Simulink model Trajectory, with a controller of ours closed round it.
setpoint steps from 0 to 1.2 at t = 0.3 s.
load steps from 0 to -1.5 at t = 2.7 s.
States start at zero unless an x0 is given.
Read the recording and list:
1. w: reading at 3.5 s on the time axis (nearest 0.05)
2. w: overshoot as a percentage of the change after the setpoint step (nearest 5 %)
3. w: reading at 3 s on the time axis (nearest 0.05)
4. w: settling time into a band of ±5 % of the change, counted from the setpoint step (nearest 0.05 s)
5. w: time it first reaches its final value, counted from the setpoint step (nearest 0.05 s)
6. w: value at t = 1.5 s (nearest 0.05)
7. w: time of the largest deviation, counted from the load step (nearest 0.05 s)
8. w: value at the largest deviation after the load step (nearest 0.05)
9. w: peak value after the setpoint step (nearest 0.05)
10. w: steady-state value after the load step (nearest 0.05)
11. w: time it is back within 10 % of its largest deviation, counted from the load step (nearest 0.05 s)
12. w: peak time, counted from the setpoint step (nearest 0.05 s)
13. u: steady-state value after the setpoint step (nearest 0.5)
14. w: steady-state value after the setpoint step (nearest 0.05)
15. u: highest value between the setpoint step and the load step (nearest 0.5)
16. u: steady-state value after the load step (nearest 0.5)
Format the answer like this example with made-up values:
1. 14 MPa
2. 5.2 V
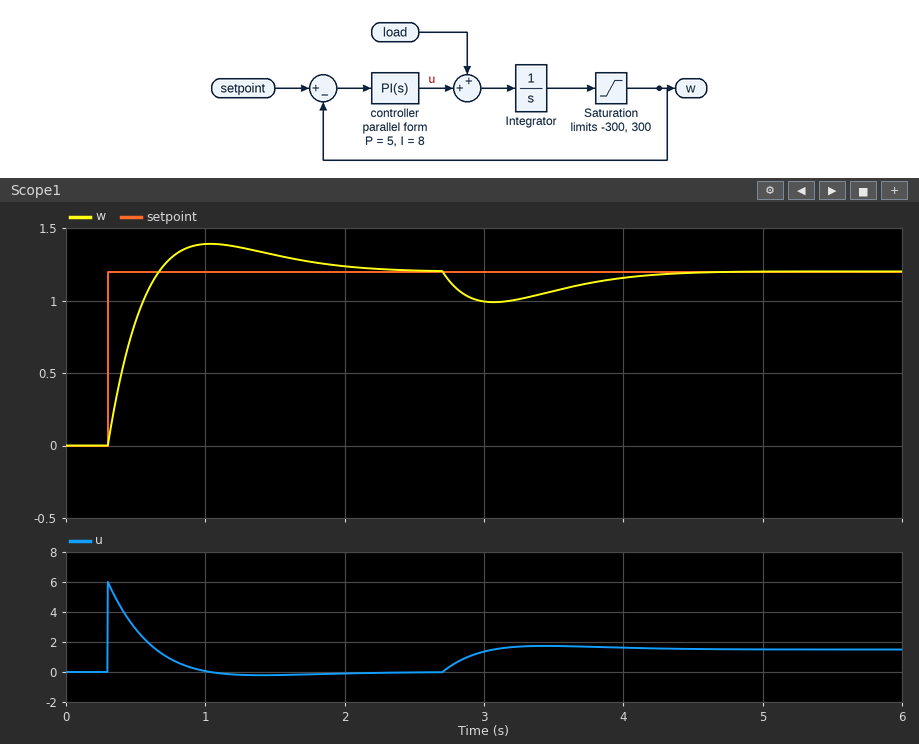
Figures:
1. 1.05
2. 15 %
3. 1.00
4. 1.50 s
5. 0.35 s
6. 1.30
7. 0.35 s
8. 1.00
9. 1.40
10. 1.20
11. 1.55 s
12. 0.75 s
13. 0.0
14. 1.20
15. 6.0
16. 1.5
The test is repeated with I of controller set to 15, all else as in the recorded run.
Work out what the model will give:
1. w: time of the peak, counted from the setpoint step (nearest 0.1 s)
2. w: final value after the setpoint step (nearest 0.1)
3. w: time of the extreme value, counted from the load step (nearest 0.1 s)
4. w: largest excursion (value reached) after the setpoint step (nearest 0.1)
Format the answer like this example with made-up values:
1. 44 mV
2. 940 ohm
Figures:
1. 0.6 s
2. 1.2
3. 0.3 s
4. 1.5
